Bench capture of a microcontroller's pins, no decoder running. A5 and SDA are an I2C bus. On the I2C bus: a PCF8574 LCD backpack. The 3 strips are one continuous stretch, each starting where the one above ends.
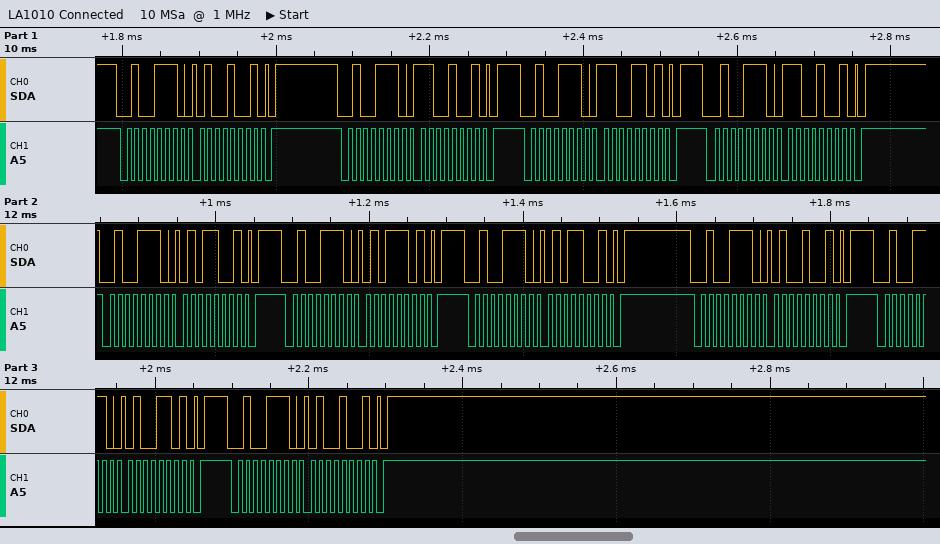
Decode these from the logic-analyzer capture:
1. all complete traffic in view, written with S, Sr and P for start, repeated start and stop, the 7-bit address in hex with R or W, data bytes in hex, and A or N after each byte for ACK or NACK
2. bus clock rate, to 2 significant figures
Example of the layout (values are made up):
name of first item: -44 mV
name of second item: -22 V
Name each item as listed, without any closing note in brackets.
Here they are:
all complete traffic in view, written with S, Sr and P for start, repeated start and stop, the 7-bit address in hex with R or W, data bytes in hex, and A or N after each byte for ACK or NACK: S 27W A 49 A P S 27W A C9 A P S 27W A CD A P S 27W A C9 A P S 27W A 59 A P S 27W A 5D A P S 27W A 59 A P S 27W A 49 A P S 27W A 4D A P S 27W A 49 A P
bus clock rate, to 2 significant figures: 100 kHz
